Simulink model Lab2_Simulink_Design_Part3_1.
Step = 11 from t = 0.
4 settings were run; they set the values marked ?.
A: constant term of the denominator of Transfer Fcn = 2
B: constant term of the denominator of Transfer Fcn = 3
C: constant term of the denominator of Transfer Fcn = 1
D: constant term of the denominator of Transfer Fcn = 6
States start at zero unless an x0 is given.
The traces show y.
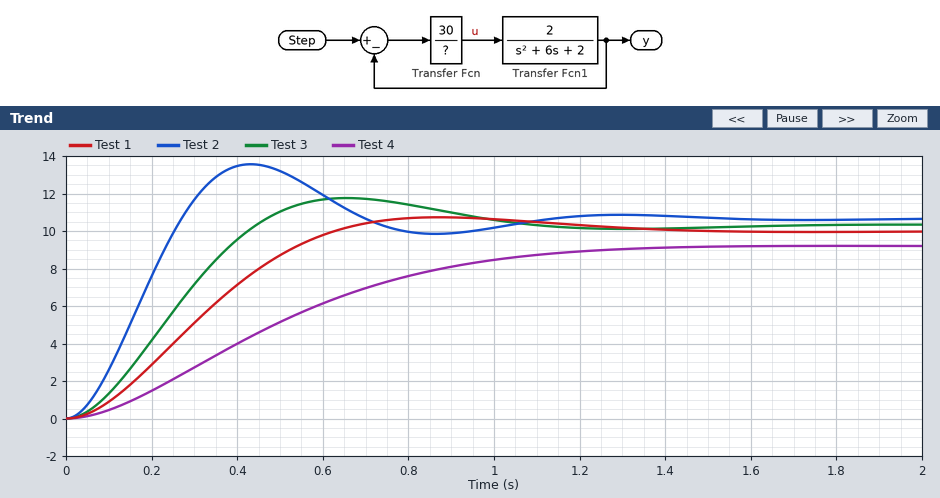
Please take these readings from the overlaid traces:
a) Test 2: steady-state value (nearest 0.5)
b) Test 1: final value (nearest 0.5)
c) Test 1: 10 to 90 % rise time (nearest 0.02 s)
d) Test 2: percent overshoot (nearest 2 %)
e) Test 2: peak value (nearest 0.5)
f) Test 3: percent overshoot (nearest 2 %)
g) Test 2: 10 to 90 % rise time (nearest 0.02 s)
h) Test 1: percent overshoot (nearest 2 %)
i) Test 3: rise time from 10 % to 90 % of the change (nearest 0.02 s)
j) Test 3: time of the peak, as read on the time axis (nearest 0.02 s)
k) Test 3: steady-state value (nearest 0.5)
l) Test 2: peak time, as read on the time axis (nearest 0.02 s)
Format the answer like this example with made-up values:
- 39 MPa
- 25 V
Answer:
- 10.5
- 10.0
- 0.42 s
- 28 %
- 13.5
- 14 %
- 0.18 s
- 8 %
- 0.30 s
- 0.66 s
- 10.5
- 0.44 s
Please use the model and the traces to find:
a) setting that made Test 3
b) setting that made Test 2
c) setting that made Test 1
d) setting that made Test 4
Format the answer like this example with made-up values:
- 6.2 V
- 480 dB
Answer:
- A
- C
- B
- D
